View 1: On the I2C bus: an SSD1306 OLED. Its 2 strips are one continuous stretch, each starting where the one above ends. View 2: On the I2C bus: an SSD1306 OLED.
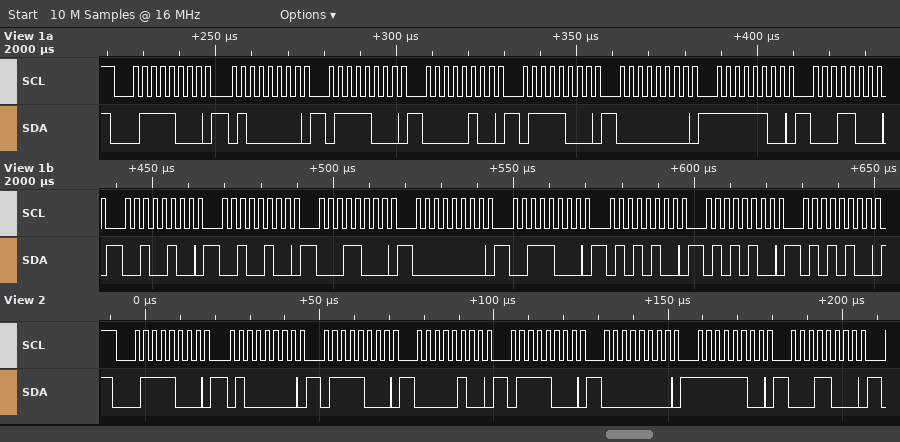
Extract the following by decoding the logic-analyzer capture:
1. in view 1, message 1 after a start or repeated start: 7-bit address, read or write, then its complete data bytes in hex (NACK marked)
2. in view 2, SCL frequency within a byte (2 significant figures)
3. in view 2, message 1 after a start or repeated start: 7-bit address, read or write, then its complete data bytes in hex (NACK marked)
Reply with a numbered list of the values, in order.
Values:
1. 0x3C write: 40 78 04 78 00 FC 18 24 24 18 00 38 54 54 54
2. 400 kHz
3. 0x3C write: 40 78 04 78 00 FC 18
